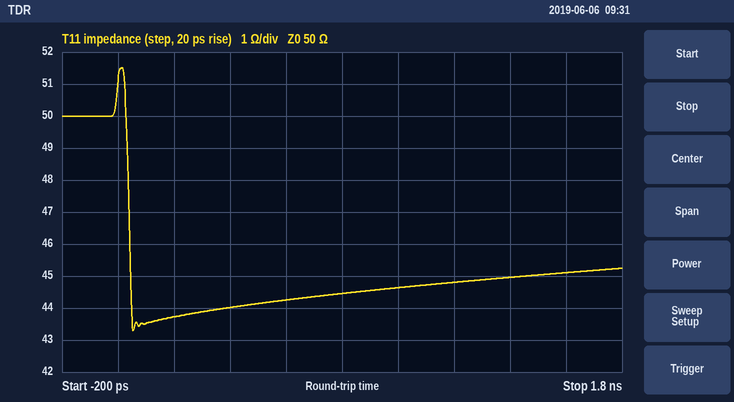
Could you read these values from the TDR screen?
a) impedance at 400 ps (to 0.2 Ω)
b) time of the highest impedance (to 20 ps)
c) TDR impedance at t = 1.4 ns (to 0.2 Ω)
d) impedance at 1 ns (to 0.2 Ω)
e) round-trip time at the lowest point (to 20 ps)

44.0 Ω
20 ps
45.0 Ω
44.6 Ω
60 ps
